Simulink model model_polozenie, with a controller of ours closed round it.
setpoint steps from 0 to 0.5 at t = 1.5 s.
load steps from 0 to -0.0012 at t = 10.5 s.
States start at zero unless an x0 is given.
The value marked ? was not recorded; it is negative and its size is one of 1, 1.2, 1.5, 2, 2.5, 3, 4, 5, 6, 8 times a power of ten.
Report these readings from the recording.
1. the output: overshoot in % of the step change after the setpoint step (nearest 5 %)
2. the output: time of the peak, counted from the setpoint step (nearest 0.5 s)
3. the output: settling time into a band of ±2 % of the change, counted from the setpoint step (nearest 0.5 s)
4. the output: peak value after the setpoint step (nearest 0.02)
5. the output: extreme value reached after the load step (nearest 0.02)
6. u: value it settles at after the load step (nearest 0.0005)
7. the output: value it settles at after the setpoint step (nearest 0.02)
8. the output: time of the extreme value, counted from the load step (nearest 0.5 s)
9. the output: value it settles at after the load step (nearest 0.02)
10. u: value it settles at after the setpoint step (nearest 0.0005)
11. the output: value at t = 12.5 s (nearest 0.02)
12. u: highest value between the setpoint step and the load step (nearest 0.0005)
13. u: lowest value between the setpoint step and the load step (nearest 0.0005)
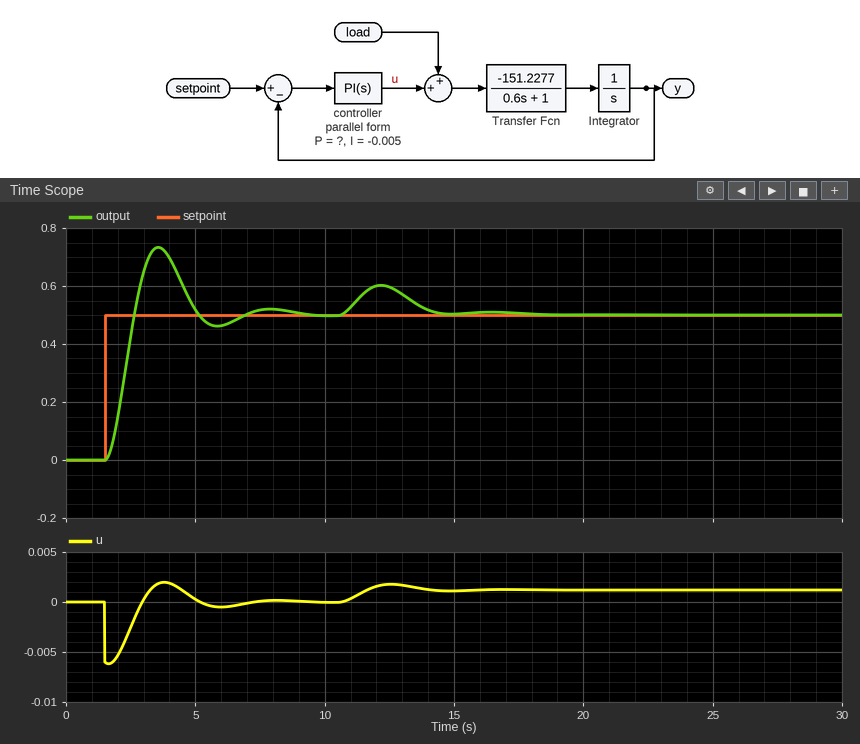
45 %
2.0 s
7.5 s
0.74
0.60
0.0010
0.50
1.5 s
0.50
0.0000
0.60
0.0020
-0.0060
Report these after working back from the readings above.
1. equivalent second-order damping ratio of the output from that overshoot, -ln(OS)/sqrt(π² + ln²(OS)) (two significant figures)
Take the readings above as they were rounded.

0.25
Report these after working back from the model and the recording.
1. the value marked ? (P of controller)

-0.012
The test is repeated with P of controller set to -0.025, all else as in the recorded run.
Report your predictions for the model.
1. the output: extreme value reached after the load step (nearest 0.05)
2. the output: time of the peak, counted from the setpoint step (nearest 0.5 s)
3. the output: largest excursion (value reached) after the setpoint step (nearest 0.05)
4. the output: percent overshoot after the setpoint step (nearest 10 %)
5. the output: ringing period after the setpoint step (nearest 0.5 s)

0.55
1.5 s
0.70
40 %
2.5 s
